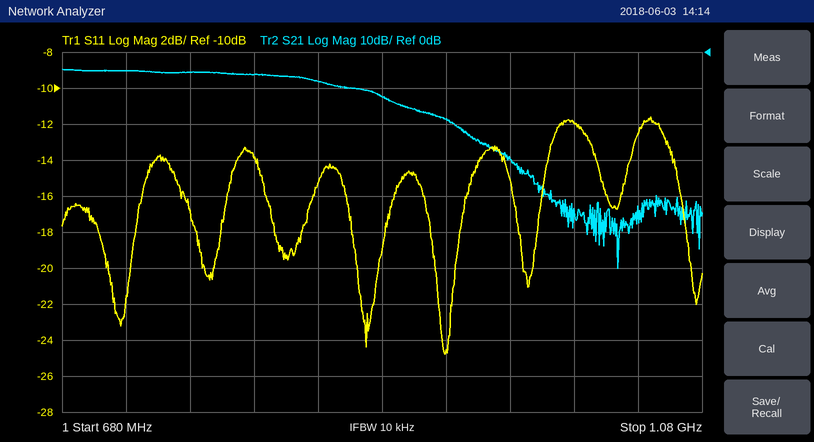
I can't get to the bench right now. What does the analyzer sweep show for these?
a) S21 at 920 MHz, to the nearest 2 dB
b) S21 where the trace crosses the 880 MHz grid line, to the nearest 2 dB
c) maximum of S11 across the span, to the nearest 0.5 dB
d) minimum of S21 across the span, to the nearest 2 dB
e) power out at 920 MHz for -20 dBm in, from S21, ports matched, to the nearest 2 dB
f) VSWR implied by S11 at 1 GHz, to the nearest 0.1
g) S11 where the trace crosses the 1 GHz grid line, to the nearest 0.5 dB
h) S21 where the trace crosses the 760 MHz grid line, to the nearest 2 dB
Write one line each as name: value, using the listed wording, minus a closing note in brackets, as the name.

S21 at 920 MHz, to the nearest 2 dB: -18 dB
S21 where the trace crosses the 880 MHz grid line, to the nearest 2 dB: -12 dB
maximum of S11 across the span, to the nearest 0.5 dB: -11.5 dB
minimum of S21 across the span, to the nearest 2 dB: -60 dB
power out at 920 MHz for -20 dBm in, from S21, ports matched, to the nearest 2 dB: -38 dBm
VSWR implied by S11 at 1 GHz, to the nearest 0.1: 1.7
S11 where the trace crosses the 1 GHz grid line, to the nearest 0.5 dB: -12.0 dB
S21 where the trace crosses the 760 MHz grid line, to the nearest 2 dB: -6 dB
